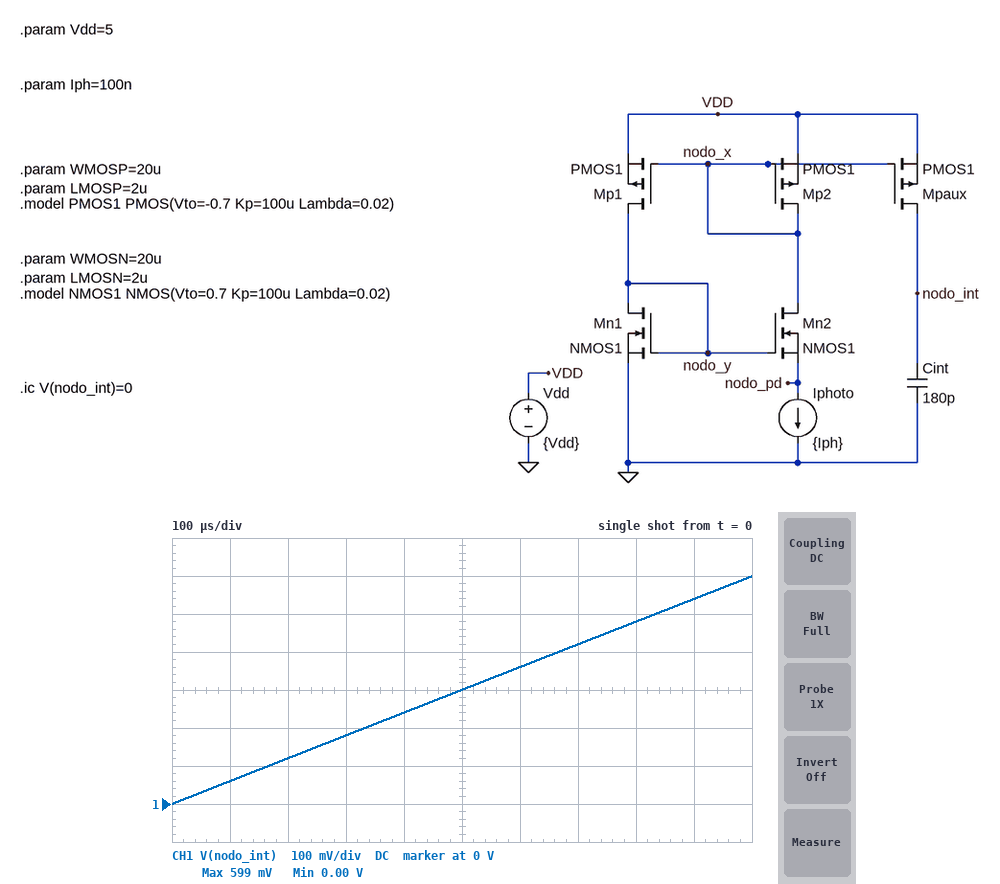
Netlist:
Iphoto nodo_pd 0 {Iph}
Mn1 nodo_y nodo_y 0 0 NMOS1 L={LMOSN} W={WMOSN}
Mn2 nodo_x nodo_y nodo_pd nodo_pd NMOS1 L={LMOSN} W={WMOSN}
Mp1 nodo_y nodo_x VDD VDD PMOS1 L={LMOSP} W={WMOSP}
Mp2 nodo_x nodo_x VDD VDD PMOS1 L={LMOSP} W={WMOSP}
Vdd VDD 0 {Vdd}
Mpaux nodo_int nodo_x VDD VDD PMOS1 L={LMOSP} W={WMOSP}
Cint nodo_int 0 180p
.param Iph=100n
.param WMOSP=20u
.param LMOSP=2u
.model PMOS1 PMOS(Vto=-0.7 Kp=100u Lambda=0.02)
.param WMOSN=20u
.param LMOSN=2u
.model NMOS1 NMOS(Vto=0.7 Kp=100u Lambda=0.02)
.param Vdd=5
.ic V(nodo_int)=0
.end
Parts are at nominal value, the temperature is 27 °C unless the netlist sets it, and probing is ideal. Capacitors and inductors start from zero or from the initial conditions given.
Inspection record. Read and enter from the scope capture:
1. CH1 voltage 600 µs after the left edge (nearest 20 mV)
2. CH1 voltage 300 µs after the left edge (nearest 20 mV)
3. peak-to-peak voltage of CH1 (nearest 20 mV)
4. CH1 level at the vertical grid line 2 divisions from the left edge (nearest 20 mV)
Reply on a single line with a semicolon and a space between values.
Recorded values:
360 mV; 180 mV; 600 mV; 120 mV
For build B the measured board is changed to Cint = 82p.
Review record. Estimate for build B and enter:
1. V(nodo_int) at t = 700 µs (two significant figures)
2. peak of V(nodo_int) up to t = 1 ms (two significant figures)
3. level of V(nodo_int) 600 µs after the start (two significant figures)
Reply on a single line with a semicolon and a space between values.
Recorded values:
920 mV; 1.3 V; 790 mV
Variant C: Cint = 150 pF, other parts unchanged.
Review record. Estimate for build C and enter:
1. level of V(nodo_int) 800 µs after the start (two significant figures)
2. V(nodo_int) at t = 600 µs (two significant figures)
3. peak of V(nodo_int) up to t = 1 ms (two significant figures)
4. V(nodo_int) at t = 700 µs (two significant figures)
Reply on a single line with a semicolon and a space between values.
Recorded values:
580 mV; 430 mV; 720 mV; 500 mV
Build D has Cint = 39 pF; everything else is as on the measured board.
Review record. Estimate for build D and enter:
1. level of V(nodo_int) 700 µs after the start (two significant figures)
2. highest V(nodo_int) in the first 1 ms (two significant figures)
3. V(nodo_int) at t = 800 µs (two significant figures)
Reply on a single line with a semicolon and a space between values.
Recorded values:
1.9 V; 2.7 V; 2.2 V
